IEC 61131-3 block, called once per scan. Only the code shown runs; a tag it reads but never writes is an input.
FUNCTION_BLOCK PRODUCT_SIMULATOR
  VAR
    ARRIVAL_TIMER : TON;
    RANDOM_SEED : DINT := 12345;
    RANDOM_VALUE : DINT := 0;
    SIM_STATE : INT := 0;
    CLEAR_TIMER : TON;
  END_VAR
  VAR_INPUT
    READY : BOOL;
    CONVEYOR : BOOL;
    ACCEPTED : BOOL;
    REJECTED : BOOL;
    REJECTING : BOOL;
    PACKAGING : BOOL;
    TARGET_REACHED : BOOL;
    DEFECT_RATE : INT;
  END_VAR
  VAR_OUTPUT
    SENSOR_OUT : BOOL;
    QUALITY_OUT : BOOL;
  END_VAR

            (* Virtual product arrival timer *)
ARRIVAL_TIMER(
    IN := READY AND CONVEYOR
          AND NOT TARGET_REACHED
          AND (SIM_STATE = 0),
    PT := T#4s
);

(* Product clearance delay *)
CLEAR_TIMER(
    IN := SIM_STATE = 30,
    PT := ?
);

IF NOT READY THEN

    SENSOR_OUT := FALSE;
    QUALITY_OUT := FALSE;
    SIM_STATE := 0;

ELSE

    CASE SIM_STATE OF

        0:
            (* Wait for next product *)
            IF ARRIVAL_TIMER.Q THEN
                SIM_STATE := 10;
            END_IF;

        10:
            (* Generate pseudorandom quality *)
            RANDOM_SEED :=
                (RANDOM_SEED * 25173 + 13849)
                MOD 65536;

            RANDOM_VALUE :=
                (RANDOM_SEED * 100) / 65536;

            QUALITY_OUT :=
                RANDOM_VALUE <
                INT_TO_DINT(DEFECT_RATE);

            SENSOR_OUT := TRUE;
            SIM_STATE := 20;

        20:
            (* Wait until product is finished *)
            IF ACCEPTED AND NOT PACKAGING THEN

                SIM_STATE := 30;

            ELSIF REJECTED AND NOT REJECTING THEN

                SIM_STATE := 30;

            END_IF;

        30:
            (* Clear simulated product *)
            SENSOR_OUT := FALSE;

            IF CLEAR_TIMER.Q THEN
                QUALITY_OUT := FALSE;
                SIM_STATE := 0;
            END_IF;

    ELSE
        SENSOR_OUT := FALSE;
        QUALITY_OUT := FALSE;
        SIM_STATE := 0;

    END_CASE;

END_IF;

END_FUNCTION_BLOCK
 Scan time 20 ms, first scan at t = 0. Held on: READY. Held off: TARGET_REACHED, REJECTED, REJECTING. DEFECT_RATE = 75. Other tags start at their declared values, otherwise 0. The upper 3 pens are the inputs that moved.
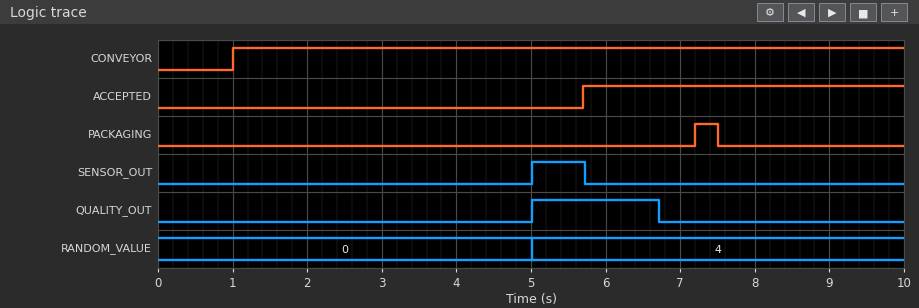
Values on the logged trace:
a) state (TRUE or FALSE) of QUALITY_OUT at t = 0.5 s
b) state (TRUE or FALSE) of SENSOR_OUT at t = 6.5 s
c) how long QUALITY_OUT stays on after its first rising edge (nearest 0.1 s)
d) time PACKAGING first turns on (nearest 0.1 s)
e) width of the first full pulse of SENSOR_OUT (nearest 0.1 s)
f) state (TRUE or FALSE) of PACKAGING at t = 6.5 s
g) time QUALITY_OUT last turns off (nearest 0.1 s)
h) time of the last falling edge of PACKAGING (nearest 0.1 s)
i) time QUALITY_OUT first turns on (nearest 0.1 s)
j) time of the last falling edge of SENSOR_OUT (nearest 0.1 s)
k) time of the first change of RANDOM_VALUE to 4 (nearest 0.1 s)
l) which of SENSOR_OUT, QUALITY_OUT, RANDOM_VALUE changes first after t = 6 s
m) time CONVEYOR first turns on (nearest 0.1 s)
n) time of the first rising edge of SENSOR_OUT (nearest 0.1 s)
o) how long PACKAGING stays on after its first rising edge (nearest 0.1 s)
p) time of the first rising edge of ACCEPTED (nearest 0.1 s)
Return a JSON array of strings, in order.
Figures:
["FALSE", "FALSE", "1.7 s", "7.2 s", "0.7 s", "FALSE", "6.7 s", "7.5 s", "5.0 s", "5.7 s", "5.0 s", "QUALITY_OUT", "1.0 s", "5.0 s", "0.3 s", "5.7 s"]
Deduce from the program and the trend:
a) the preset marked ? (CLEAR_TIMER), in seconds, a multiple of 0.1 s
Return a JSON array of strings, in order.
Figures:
["1.0 s"]
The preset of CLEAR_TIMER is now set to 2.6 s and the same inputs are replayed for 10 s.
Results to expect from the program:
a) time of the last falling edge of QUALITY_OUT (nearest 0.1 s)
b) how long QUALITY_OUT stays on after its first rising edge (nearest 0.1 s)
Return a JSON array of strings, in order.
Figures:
["8.3 s", "3.3 s"]
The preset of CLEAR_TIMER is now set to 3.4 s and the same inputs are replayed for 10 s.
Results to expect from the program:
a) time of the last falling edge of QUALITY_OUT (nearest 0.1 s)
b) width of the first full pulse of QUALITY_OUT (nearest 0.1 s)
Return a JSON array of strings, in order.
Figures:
["9.1 s", "4.1 s"]
